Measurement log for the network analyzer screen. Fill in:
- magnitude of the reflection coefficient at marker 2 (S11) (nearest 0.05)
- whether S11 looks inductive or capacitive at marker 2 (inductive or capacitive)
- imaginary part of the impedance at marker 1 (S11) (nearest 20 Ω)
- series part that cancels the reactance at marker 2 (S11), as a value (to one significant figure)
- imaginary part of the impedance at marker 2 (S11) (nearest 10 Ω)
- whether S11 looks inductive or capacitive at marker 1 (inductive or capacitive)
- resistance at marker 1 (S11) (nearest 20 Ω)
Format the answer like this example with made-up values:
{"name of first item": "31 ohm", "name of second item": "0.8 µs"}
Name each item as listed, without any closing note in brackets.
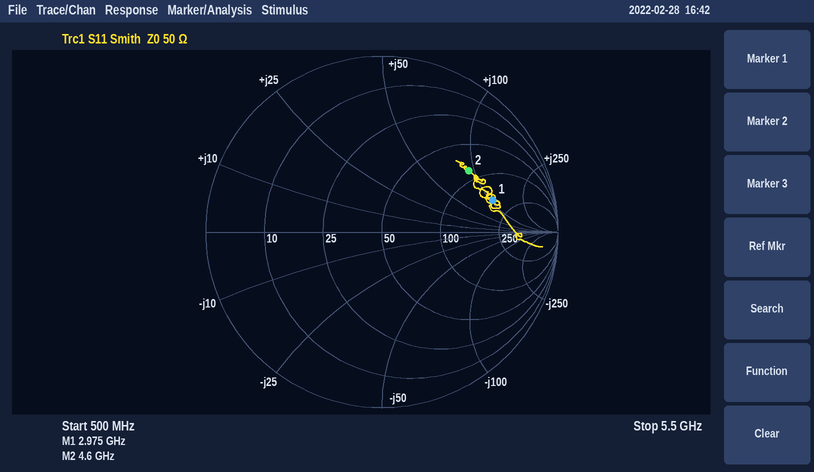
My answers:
{"magnitude of the reflection coefficient at marker 2 (S11)": "0.60", "whether S11 looks inductive or capacitive at marker 2": "inductive", "imaginary part of the impedance at marker 1 (S11)": "+100 Ω", "series part that cancels the reactance at marker 2 (S11), as a value": "400 fF", "imaginary part of the impedance at marker 2 (S11)": "+90 Ω", "whether S11 looks inductive or capacitive at marker 1": "inductive", "resistance at marker 1 (S11)": "160 Ω"}
